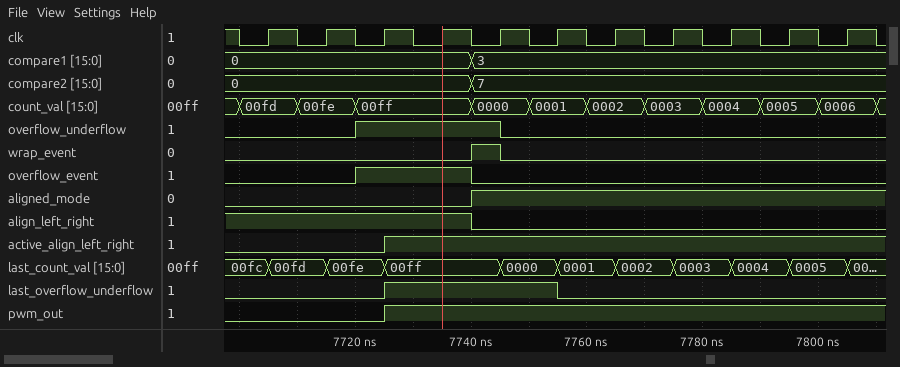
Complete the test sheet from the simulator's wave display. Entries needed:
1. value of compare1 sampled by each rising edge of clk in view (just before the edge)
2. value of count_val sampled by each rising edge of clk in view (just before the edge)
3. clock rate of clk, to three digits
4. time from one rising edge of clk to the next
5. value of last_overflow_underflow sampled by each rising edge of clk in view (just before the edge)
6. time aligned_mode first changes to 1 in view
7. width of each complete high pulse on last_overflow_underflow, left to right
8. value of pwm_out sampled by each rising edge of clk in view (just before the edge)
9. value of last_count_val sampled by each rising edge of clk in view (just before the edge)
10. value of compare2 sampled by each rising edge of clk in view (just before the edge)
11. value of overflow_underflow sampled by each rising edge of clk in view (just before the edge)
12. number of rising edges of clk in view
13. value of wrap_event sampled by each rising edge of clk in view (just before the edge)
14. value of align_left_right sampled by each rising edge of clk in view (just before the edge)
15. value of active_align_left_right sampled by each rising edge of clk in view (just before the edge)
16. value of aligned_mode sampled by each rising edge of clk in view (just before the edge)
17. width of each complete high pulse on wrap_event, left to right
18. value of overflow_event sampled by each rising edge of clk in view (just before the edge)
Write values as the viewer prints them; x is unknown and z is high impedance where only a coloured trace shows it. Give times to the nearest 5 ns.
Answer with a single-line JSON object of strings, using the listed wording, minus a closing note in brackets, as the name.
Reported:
{"value of compare1 sampled by each rising edge of clk in view": "0, 0, 0, 0, 3, 3, 3, 3, 3, 3, 3", "value of count_val sampled by each rising edge of clk in view": "00fd, 00fe, 00ff, 00ff, 0000, 0001, 0002, 0003, 0004, 0005, 0006", "clock rate of clk, to three digits": "100 MHz", "time from one rising edge of clk to the next": "10 ns", "value of last_overflow_underflow sampled by each rising edge of clk in view": "0 0 0 1 1 1 0 0 0 0 0", "time aligned_mode first changes to 1 in view": "7740 ns", "width of each complete high pulse on last_overflow_underflow, left to right": "30 ns", "value of pwm_out sampled by each rising edge of clk in view": "0 0 0 1 1 1 1 1 1 1 1", "value of last_count_val sampled by each rising edge of clk in view": "00fc, 00fd, 00fe, 00ff, 00ff, 0000, 0001, 0002, 0003, 0004, 0005", "value of compare2 sampled by each rising edge of clk in view": "0, 0, 0, 0, 7, 7, 7, 7, 7, 7, 7", "value of overflow_underflow sampled by each rising edge of clk in view": "0 0 1 1 1 0 0 0 0 0 0", "number of rising edges of clk in view": "11", "value of wrap_event sampled by each rising edge of clk in view": "0 0 0 0 1 0 0 0 0 0 0", "value of align_left_right sampled by each rising edge of clk in view": "1 1 1 1 0 0 0 0 0 0 0", "value of active_align_left_right sampled by each rising edge of clk in view": "0 0 0 1 1 1 1 1 1 1 1", "value of aligned_mode sampled by each rising edge of clk in view": "0 0 0 0 1 1 1 1 1 1 1", "width of each complete high pulse on wrap_event, left to right": "5 ns", "value of overflow_event sampled by each rising edge of clk in view": "0 0 1 1 0 0 0 0 0 0 0"}
